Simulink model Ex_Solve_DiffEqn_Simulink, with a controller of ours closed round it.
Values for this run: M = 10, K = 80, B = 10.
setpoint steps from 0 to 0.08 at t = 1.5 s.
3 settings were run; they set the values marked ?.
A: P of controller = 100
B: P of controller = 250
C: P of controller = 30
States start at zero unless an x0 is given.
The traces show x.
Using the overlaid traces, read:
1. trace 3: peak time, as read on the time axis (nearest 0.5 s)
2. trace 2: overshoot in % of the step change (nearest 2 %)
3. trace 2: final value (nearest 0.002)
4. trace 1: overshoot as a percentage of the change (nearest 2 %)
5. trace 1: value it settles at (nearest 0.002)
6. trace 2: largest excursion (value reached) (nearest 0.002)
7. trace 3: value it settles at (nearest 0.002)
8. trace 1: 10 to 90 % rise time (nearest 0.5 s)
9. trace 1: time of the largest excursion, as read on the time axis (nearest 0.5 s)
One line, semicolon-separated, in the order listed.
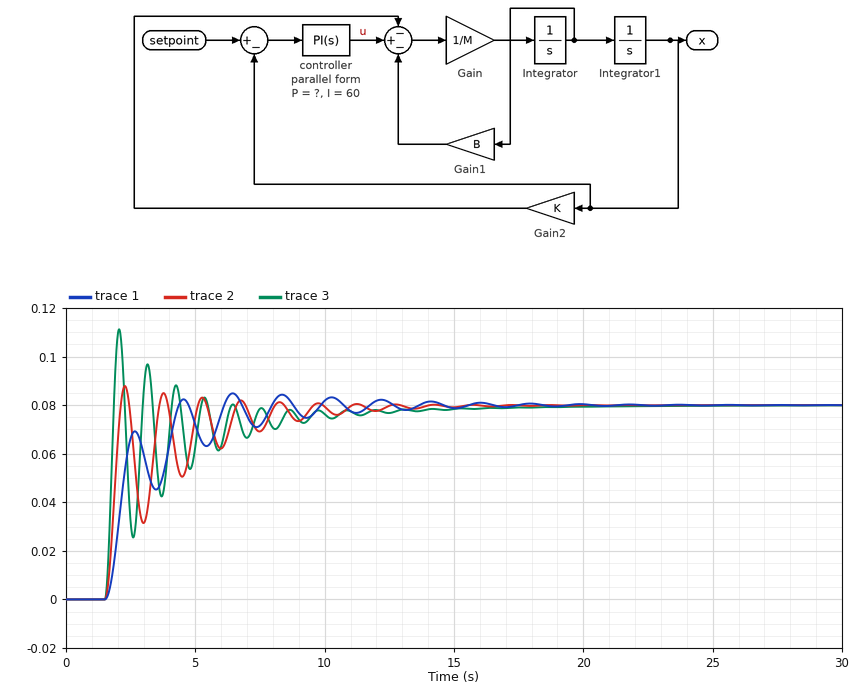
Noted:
2.0 s; 10 %; 0.080; 6 %; 0.080; 0.088; 0.080; 2.5 s; 6.5 s
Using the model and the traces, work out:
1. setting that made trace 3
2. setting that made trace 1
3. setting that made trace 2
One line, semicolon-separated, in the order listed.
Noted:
B; C; A
